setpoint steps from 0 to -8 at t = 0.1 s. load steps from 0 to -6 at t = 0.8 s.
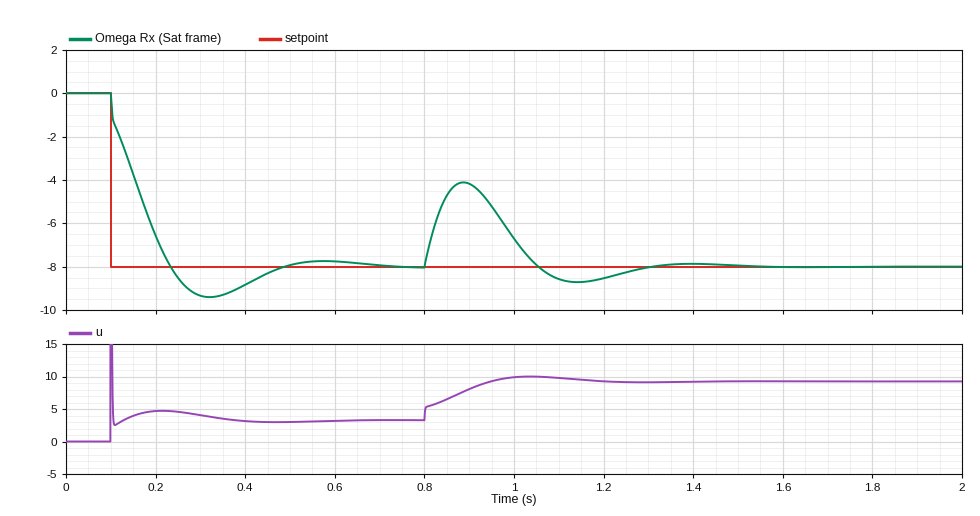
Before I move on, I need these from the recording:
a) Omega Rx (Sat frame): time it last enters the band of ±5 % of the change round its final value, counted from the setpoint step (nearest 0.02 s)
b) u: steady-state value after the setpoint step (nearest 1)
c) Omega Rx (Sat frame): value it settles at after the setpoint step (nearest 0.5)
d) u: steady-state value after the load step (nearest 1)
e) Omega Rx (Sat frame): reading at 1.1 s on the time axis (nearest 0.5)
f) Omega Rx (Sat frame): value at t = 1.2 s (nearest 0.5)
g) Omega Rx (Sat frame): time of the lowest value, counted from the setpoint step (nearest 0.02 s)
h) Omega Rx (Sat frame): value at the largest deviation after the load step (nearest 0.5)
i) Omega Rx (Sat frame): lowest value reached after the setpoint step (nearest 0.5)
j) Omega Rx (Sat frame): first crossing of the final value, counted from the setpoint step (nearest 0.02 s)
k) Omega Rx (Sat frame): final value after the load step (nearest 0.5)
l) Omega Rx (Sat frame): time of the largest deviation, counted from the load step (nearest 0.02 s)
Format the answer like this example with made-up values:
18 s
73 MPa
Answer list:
0.34 s
3
-8.0
9
-8.5
-8.5
0.22 s
-4.0
-9.5
0.14 s
-8.0
0.08 s
